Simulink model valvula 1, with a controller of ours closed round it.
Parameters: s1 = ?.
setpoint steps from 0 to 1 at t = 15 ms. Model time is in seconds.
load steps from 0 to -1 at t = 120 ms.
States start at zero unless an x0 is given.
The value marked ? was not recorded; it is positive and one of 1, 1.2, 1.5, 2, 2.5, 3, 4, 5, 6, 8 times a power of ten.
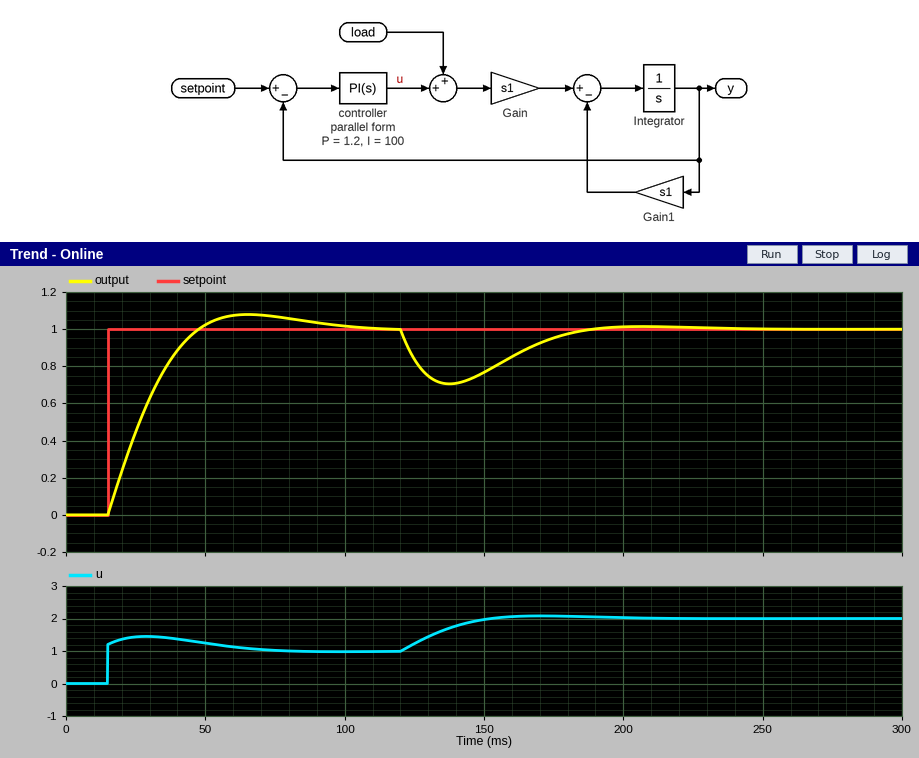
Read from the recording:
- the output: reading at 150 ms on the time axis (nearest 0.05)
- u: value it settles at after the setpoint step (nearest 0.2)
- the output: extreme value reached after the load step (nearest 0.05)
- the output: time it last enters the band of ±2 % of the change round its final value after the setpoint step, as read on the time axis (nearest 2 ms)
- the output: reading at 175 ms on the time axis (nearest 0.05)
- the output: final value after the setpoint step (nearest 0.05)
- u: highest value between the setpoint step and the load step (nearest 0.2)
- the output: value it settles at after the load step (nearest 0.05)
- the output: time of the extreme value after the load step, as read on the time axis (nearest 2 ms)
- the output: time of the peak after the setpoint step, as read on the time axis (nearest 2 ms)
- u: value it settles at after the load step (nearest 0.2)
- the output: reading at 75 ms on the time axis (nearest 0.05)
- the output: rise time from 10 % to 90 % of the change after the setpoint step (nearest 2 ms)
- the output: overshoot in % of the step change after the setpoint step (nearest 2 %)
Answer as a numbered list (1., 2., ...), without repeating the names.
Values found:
1. 0.75
2. 1.0
3. 0.70
4. 98 ms
5. 0.95
6. 1.00
7. 1.4
8. 1.00
9. 138 ms
10. 66 ms
11. 2.0
12. 1.05
13. 24 ms
14. 8 %
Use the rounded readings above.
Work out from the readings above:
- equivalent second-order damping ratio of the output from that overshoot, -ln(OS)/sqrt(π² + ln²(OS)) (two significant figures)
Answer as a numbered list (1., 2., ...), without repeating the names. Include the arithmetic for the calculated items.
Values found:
1. ln(0.08) = -2.526; 2.526 / sqrt(9.870 + 6.379) = 0.63
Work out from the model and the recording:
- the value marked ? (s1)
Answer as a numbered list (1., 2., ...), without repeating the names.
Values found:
1. 40
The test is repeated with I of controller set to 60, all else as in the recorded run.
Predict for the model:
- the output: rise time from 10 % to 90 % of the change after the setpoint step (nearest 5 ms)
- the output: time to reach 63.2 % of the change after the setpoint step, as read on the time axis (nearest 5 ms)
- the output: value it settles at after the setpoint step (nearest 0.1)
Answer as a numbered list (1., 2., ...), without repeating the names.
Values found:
1. 35 ms
2. 35 ms
3. 1.0
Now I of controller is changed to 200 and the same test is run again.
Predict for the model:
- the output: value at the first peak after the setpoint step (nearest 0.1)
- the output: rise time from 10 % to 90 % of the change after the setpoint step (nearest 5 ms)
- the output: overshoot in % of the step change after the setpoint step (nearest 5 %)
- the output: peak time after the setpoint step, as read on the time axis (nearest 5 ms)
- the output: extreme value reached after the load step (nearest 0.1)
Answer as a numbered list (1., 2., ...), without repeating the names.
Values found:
1. 1.2
2. 15 ms
3. 20 %
4. 50 ms
5. 0.8
